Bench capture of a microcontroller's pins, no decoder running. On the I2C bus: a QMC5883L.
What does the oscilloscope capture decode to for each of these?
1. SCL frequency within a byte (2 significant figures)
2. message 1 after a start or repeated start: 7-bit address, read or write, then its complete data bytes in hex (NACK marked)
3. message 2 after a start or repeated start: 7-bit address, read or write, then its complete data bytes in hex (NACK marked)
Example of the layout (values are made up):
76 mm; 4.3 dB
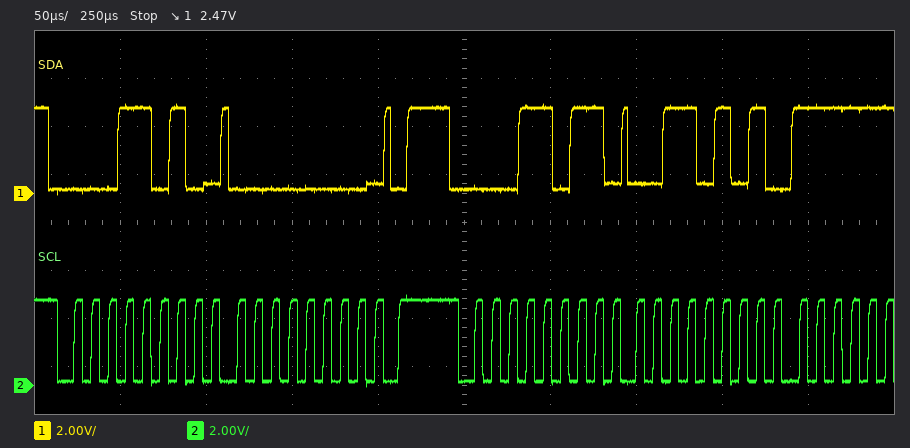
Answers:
100 kHz; 0x0D write: 00; 0x0D read: 35
